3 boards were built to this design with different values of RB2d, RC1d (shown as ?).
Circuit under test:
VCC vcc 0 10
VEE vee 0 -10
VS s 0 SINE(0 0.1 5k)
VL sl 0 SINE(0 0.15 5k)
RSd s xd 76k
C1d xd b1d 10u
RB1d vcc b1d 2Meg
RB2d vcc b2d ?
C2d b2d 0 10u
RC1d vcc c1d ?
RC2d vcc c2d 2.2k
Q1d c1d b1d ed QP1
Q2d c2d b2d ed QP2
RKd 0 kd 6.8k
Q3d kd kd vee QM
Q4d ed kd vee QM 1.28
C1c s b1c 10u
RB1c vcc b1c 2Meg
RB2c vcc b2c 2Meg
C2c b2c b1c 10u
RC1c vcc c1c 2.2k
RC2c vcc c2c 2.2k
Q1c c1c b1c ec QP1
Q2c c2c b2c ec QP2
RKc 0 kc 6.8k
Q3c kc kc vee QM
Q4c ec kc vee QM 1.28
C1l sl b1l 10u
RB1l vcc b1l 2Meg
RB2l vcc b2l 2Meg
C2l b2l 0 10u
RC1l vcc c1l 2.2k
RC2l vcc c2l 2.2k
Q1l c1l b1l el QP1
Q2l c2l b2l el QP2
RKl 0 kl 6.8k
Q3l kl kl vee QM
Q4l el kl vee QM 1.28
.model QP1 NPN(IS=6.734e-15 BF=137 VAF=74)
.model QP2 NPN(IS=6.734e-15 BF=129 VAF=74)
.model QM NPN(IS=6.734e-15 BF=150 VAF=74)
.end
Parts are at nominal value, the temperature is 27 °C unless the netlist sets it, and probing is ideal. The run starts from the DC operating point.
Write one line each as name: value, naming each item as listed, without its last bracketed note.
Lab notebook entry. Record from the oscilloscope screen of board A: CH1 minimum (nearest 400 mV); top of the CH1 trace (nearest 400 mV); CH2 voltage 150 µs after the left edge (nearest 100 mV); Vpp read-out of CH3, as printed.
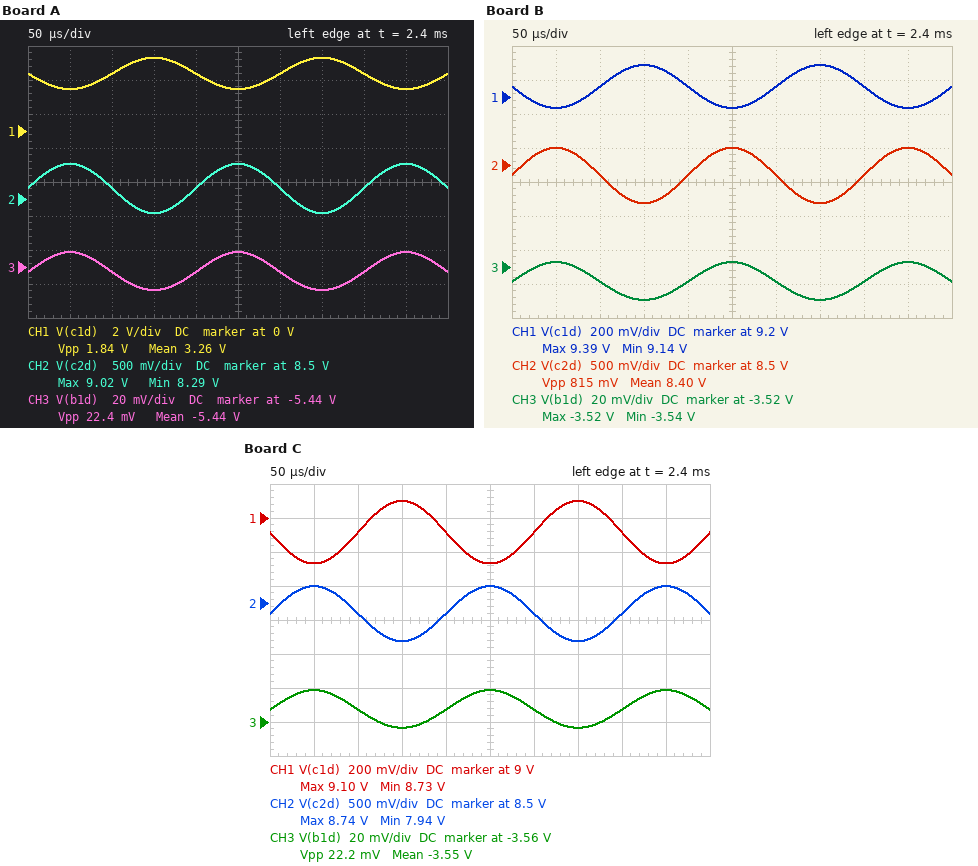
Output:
CH1 minimum: 2.4 V
top of the CH1 trace: 4.4 V
CH2 voltage 150 µs after the left edge: 8.3 V
Vpp read-out of CH3, as printed: 22.4 mV
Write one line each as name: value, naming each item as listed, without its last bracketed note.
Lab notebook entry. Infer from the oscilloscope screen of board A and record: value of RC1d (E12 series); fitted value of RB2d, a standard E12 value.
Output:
value of RC1d: 5.6 kΩ
fitted value of RB2d, a standard E12 value: 3.9 MΩ
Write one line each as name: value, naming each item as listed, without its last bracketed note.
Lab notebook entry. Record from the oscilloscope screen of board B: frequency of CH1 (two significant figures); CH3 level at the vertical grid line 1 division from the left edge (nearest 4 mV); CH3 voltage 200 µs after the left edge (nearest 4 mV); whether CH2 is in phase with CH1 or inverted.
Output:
frequency of CH1: 5.0 kHz
CH3 level at the vertical grid line 1 division from the left edge: -3.516 V
CH3 voltage 200 µs after the left edge: -3.528 V
whether CH2 is in phase with CH1 or inverted: inverted
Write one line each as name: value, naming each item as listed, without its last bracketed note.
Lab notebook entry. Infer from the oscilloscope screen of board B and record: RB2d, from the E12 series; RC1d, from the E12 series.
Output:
RB2d, from the E12 series: 2.7 MΩ
RC1d, from the E12 series: 680 Ω
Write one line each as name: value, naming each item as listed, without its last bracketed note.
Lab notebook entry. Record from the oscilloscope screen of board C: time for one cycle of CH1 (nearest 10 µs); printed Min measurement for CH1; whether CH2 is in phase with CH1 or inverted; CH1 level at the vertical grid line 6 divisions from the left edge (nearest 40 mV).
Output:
time for one cycle of CH1: 200 µs
printed Min measurement for CH1: 8.73 V
whether CH2 is in phase with CH1 or inverted: inverted
CH1 level at the vertical grid line 6 divisions from the left edge: 8.92 V
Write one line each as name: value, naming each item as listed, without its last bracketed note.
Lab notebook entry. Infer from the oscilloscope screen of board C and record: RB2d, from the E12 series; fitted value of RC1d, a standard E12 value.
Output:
RB2d, from the E12 series: 2.7 MΩ
fitted value of RC1d, a standard E12 value: 1 kΩ
